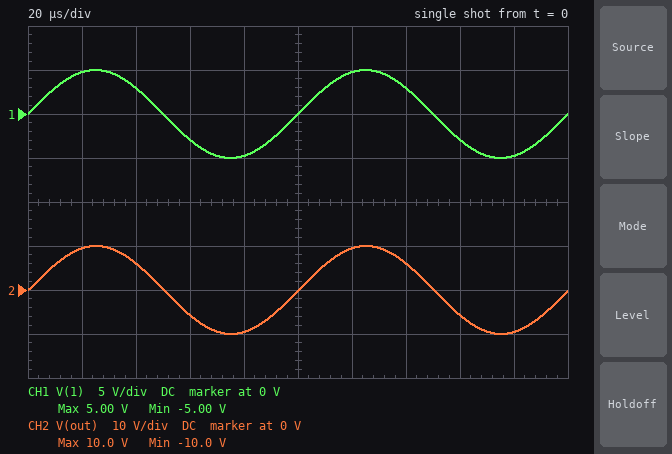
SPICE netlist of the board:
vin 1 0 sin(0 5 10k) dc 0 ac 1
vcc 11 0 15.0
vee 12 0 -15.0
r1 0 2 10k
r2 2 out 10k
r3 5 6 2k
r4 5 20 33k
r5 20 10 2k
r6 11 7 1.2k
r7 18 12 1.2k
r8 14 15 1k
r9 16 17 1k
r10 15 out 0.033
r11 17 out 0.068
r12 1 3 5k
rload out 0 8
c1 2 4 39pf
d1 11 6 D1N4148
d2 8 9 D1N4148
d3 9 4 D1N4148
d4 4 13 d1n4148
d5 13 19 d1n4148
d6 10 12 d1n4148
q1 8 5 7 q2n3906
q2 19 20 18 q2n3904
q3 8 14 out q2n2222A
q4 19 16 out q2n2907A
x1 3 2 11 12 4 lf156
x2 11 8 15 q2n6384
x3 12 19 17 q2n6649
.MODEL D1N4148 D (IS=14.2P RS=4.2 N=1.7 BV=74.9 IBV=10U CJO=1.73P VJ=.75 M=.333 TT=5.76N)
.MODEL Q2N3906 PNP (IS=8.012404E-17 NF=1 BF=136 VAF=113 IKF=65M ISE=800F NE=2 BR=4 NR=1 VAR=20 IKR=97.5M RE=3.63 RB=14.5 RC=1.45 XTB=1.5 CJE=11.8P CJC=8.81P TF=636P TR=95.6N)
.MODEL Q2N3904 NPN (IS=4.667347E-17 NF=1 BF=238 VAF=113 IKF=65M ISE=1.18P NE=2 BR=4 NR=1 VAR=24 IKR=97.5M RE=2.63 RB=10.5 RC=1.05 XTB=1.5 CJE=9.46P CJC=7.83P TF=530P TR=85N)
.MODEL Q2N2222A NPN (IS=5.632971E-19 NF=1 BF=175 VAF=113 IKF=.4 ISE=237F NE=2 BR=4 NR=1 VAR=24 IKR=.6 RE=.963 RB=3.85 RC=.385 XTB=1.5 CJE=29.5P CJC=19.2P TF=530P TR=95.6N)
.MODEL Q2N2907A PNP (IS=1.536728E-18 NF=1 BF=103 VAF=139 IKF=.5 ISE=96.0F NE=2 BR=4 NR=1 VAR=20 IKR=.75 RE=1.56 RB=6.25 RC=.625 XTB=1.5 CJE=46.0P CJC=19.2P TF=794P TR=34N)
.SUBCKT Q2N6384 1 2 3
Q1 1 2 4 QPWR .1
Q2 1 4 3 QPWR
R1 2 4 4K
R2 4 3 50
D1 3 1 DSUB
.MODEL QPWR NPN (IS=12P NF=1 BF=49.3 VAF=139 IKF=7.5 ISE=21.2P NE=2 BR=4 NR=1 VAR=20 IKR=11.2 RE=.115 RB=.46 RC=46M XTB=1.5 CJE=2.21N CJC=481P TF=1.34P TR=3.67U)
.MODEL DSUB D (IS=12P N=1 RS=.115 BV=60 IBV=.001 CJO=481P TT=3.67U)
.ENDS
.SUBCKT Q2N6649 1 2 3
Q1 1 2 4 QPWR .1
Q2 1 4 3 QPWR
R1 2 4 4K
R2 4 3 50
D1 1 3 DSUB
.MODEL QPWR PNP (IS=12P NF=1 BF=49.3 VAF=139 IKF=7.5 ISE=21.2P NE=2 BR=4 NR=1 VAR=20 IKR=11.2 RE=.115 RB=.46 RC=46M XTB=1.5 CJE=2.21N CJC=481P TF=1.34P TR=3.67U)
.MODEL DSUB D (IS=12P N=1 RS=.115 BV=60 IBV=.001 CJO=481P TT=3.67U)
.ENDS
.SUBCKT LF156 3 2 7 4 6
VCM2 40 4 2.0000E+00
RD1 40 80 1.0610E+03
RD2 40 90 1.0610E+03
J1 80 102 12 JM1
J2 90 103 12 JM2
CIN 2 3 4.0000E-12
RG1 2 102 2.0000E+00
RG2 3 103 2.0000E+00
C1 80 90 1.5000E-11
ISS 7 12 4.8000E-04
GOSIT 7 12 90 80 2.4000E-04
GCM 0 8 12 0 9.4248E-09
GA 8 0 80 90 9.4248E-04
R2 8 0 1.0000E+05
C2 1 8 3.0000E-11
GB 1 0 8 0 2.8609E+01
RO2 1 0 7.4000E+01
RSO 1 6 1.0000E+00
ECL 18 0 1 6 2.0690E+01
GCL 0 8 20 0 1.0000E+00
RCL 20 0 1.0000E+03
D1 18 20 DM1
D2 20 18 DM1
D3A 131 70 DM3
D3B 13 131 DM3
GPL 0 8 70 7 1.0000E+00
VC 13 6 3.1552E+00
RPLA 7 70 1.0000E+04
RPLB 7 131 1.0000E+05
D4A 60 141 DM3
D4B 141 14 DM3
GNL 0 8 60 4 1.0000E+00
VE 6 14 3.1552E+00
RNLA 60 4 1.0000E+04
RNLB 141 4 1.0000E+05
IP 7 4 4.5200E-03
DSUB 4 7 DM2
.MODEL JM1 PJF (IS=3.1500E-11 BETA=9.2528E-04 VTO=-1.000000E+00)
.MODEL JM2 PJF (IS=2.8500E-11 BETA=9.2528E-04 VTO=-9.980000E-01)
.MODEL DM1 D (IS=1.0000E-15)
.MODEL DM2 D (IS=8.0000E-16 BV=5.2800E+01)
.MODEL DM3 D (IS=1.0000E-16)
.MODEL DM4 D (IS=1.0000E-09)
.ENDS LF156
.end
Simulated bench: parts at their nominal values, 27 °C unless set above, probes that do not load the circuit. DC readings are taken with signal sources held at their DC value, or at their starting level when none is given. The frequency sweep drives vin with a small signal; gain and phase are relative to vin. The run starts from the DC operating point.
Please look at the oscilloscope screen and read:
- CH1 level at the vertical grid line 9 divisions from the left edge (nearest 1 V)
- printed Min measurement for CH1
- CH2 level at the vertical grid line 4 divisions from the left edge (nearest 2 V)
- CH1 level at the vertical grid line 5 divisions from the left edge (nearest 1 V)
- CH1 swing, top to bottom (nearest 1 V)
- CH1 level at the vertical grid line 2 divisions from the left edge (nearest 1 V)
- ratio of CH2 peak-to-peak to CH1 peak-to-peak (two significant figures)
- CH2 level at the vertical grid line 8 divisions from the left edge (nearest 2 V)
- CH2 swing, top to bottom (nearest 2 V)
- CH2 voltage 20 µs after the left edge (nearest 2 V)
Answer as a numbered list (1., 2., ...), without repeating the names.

1. -5 V
2. -5.00 V
3. -10 V
4. 0 V
5. 10 V
6. 3 V
7. 2.0
8. -6 V
9. 20 V
10. 10 V
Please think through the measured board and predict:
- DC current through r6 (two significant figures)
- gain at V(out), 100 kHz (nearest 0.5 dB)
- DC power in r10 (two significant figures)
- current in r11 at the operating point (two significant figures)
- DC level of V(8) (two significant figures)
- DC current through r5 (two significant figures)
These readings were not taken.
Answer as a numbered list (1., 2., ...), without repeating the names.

1. 1.3 mA
2. 6.0 dB
3. 36 mW
4. 1.0 A
5. 1.5 V
6. 760 µA
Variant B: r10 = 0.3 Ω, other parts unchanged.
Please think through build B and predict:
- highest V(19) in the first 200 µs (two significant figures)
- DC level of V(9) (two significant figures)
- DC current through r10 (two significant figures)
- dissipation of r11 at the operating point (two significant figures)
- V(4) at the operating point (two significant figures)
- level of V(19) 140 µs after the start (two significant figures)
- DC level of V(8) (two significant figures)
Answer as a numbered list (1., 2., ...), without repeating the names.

1. 8.9 V
2. 860 mV
3. 770 mA
4. 40 mW
5. 93 mV
6. 4.7 V
7. 1.6 V
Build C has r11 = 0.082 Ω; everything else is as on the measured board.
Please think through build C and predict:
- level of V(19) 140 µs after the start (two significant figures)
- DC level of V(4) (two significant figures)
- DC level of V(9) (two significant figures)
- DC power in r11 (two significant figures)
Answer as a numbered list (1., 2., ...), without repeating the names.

1. 4.6 V
2. -22 mV
3. 730 mV
4. 86 mW
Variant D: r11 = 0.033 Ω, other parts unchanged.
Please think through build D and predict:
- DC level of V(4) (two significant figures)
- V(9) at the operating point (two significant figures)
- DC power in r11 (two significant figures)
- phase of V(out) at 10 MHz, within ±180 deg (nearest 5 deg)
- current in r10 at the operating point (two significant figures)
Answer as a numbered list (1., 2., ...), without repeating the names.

1. 3.1 mV
2. 750 mV
3. 39 mW
4. 130 deg
5. 1.1 A
